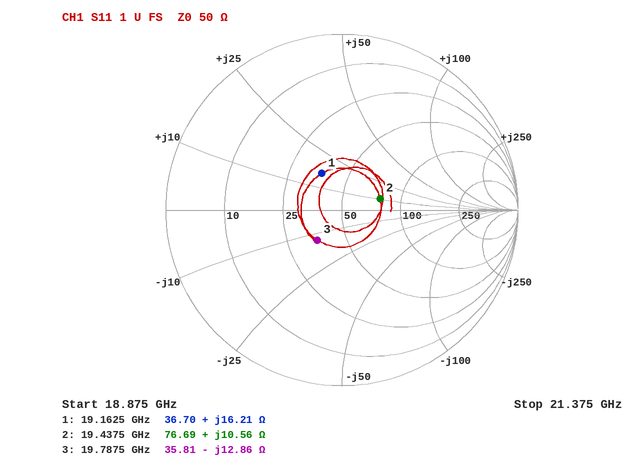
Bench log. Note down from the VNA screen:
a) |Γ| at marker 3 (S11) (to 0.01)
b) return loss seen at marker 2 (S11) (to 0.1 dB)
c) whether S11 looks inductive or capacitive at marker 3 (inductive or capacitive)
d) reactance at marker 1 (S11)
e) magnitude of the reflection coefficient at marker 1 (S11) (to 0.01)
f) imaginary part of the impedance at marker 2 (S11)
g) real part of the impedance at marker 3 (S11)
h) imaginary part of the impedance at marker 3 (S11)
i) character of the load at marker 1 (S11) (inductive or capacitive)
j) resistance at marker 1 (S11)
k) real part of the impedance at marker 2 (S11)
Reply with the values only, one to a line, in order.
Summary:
0.22
12.9 dB
capacitive
+16.21 Ω
0.24
+10.56 Ω
35.81 Ω
-12.86 Ω
inductive
36.70 Ω
76.69 Ω
